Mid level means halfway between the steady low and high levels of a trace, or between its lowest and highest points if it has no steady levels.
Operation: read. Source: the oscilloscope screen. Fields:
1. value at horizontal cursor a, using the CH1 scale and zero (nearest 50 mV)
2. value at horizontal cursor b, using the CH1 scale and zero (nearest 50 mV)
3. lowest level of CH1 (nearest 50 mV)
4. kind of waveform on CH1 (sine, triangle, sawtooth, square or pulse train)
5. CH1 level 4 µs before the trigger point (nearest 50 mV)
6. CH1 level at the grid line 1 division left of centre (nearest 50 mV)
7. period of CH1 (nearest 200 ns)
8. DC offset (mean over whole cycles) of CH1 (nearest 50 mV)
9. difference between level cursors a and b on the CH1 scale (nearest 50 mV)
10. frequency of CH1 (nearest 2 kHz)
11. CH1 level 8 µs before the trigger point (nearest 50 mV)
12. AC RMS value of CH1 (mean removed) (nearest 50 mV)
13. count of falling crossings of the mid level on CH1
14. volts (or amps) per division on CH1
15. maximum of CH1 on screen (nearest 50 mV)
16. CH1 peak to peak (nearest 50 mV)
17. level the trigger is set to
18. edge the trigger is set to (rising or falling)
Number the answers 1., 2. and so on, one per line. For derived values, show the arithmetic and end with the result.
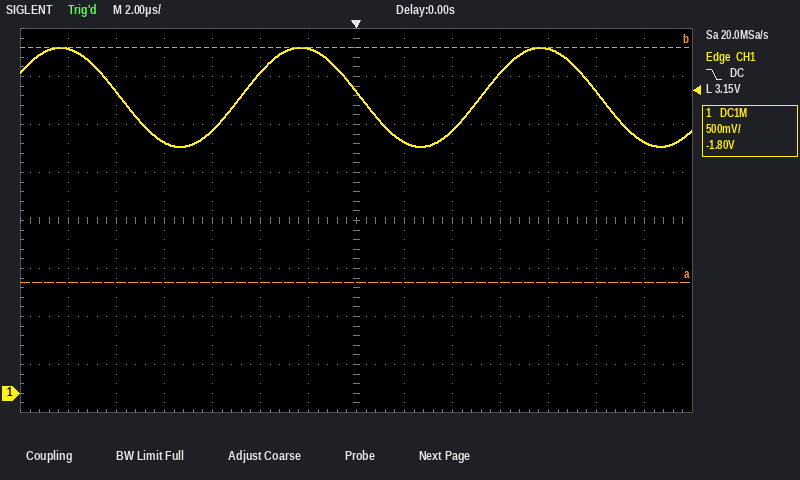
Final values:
1. 1.15 V
2. 3.60 V
3. 2.55 V
4. sine
5. 3.35 V
6. 3.60 V
7. 10.0 µs
8. (3.60 V + (2.55 V)) / 2 ≈ 3.08 V, so 3.10 V to the nearest 50 mV
9. 2.45 V
10. 1 / 10.0 µs ≈ 100 kHz
11. 2.60 V
12. 1.05 V / (2√2) ≈ 371 mV, so 350 mV to the nearest 50 mV
13. 3
14. 500 mV
15. 3.60 V
16. 3.60 V − (2.55 V) = 1.05 V
17. 3.15 V
18. falling
